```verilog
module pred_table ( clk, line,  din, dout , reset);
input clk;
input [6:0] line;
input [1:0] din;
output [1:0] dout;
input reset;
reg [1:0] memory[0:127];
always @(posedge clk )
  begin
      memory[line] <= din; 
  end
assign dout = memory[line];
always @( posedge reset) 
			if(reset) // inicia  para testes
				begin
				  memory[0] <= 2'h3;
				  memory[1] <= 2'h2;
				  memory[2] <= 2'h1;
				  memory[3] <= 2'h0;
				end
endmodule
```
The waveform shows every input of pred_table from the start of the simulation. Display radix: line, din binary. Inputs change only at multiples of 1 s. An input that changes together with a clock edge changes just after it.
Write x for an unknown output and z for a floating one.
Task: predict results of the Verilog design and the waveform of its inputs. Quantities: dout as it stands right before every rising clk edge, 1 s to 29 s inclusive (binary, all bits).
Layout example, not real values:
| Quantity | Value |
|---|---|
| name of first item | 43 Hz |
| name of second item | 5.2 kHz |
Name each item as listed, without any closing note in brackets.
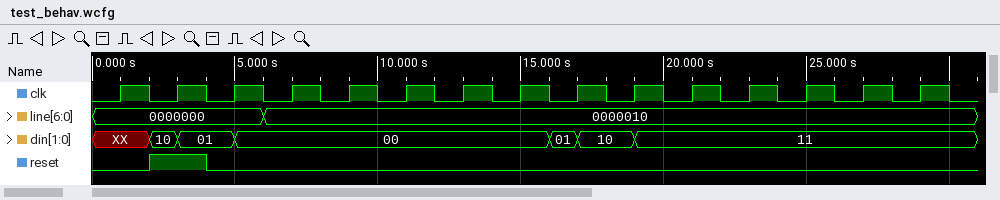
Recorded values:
| Quantity | Value |
|---|---|
| dout as it stands right before every rising clk edge, 1 s to 29 s inclusive | x, 11, 10, 01, 00, 00, 00, 00, 00, 01, 10, 11, 11, 11, 11 |
